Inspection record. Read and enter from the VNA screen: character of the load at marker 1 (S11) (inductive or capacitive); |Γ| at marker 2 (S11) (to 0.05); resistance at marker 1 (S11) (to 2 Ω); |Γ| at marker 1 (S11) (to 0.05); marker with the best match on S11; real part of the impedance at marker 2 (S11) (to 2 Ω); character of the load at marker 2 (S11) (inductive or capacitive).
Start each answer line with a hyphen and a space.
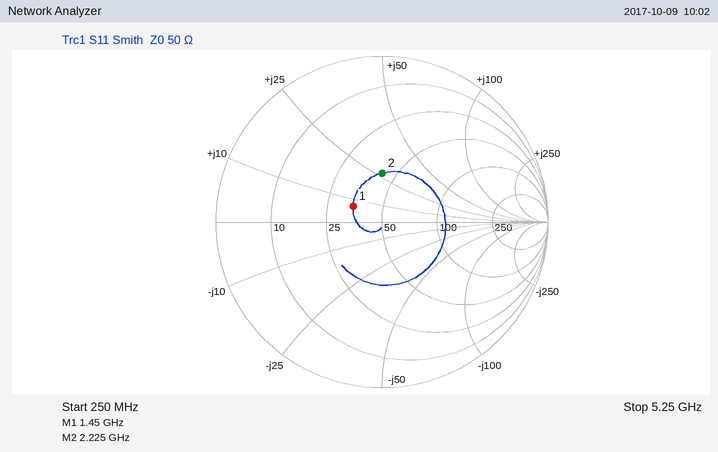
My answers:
- inductive
- 0.30
- 34 Ω
- 0.20
- marker 1
- 42 Ω
- inductive
